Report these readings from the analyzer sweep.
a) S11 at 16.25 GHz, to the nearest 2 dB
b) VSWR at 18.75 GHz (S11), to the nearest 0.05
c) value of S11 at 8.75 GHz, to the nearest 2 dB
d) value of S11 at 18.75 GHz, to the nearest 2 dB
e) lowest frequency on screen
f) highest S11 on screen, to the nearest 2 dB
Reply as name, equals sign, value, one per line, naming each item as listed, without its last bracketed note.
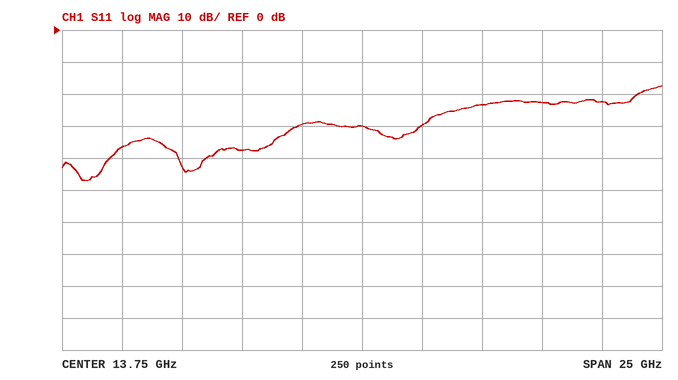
S11 at 16.25 GHz, to the nearest 2 dB = -30 dB
VSWR at 18.75 GHz (S11), to the nearest 0.05 = 1.15
value of S11 at 8.75 GHz, to the nearest 2 dB = -38 dB
value of S11 at 18.75 GHz, to the nearest 2 dB = -24 dB
lowest frequency on screen = 1.25 GHz
highest S11 on screen, to the nearest 2 dB = -18 dB
